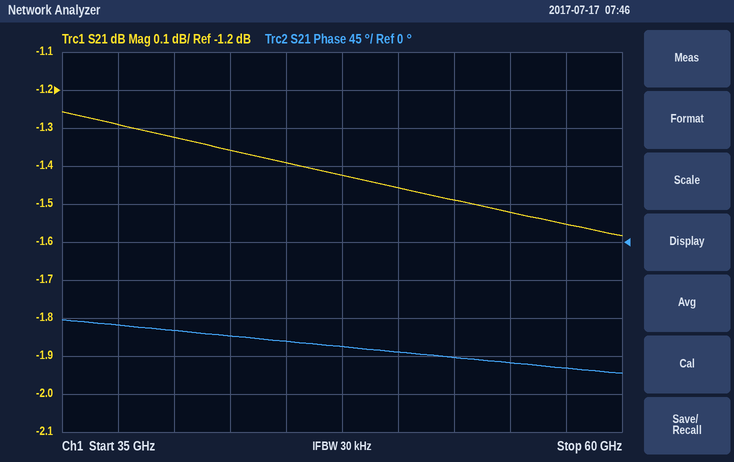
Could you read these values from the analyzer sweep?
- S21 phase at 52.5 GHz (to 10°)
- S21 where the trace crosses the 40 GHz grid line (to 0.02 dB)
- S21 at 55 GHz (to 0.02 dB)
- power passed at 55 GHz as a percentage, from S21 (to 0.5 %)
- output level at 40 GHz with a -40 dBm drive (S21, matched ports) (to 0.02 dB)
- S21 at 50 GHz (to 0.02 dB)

-140°
-1.32 dB
-1.52 dB
70.5 %
-41.32 dBm
-1.46 dB
